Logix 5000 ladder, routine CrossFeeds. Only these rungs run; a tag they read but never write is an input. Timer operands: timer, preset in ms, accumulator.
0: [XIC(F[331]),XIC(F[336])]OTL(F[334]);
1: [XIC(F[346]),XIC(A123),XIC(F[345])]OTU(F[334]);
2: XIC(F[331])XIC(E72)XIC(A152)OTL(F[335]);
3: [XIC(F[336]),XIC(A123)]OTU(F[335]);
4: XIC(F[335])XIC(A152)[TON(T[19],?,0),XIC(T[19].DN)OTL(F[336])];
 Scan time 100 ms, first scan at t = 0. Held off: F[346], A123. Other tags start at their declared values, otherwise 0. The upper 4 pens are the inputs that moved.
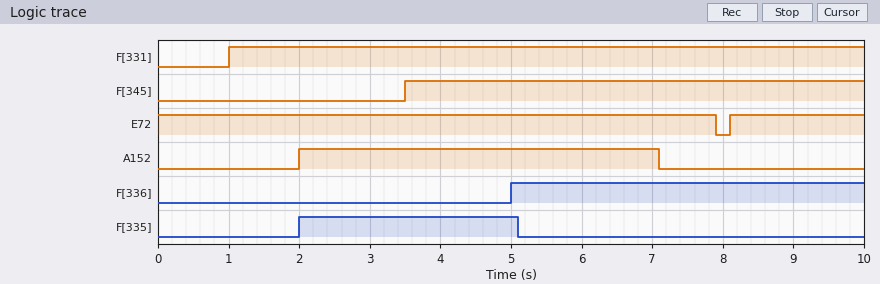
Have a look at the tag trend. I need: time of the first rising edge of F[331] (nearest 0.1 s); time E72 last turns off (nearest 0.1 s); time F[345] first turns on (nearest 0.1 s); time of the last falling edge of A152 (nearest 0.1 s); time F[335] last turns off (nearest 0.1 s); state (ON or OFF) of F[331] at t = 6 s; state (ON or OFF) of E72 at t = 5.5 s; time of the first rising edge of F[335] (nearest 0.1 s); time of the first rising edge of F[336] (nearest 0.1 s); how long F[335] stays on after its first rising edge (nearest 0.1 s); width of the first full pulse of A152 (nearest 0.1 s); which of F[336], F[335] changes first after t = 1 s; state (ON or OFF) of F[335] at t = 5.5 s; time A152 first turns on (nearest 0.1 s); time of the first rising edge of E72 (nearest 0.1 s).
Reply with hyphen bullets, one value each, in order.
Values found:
- 1.0 s
- 7.9 s
- 3.5 s
- 7.1 s
- 5.1 s
- ON
- ON
- 2.0 s
- 5.0 s
- 3.1 s
- 5.1 s
- F[335]
- OFF
- 2.0 s
- 8.1 s
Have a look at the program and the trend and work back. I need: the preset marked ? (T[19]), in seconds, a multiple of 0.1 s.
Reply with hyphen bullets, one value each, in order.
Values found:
- 3.0 s
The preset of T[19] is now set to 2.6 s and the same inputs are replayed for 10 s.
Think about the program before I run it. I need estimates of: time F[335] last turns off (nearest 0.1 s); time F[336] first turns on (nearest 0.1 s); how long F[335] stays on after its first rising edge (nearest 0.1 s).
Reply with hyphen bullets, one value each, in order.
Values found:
- 4.7 s
- 4.6 s
- 2.7 s
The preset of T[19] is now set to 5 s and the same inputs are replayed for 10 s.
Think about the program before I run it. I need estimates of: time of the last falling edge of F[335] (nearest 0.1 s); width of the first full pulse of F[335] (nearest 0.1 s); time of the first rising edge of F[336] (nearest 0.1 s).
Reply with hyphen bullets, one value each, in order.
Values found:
- 7.1 s
- 5.1 s
- 7.0 s
